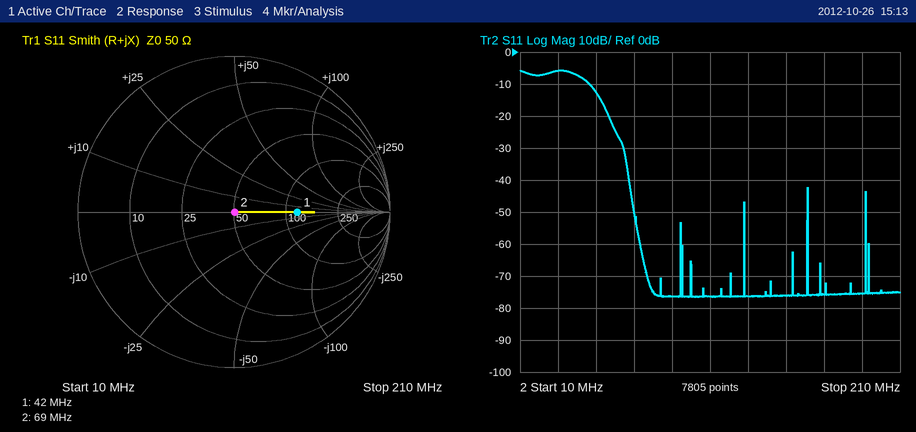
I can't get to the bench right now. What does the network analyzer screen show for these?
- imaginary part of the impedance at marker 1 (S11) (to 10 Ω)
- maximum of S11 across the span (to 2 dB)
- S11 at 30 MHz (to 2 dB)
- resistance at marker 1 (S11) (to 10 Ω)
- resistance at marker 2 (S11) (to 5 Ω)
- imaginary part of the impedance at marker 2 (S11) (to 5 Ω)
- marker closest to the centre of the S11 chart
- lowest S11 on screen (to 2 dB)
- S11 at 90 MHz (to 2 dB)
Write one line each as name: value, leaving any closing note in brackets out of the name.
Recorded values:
imaginary part of the impedance at marker 1 (S11): 0 Ω
maximum of S11 across the span: -6 dB
S11 at 30 MHz: -6 dB
resistance at marker 1 (S11): 120 Ω
resistance at marker 2 (S11): 50 Ω
imaginary part of the impedance at marker 2 (S11): 0 Ω
marker closest to the centre of the S11 chart: marker 2
lowest S11 on screen: -76 dB
S11 at 90 MHz: -76 dB
